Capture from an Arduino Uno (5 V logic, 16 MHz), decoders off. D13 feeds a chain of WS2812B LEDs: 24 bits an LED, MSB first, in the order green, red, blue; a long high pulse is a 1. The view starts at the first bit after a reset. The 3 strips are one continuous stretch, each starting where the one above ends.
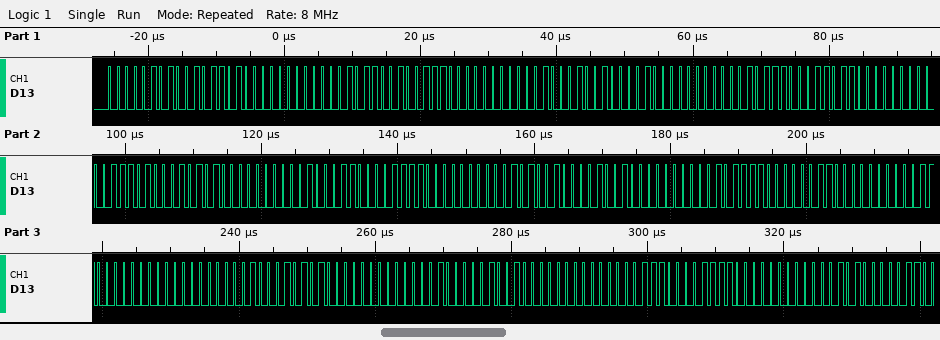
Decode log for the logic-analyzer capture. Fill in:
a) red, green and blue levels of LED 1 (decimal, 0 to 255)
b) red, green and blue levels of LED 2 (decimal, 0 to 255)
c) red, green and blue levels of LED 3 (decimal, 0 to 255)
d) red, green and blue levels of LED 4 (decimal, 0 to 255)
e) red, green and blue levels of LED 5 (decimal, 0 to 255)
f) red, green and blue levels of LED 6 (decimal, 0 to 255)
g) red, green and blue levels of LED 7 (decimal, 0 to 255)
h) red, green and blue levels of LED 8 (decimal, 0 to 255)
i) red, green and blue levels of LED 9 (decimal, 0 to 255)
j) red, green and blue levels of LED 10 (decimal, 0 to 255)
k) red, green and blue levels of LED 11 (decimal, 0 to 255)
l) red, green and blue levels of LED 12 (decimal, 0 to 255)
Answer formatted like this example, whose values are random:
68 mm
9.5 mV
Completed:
45, 5, 0
39, 11, 0
33, 17, 0
27, 23, 0
21, 29, 0
15, 35, 0
9, 41, 0
3, 47, 0
0, 48, 2
0, 42, 8
0, 36, 14
0, 30, 20
